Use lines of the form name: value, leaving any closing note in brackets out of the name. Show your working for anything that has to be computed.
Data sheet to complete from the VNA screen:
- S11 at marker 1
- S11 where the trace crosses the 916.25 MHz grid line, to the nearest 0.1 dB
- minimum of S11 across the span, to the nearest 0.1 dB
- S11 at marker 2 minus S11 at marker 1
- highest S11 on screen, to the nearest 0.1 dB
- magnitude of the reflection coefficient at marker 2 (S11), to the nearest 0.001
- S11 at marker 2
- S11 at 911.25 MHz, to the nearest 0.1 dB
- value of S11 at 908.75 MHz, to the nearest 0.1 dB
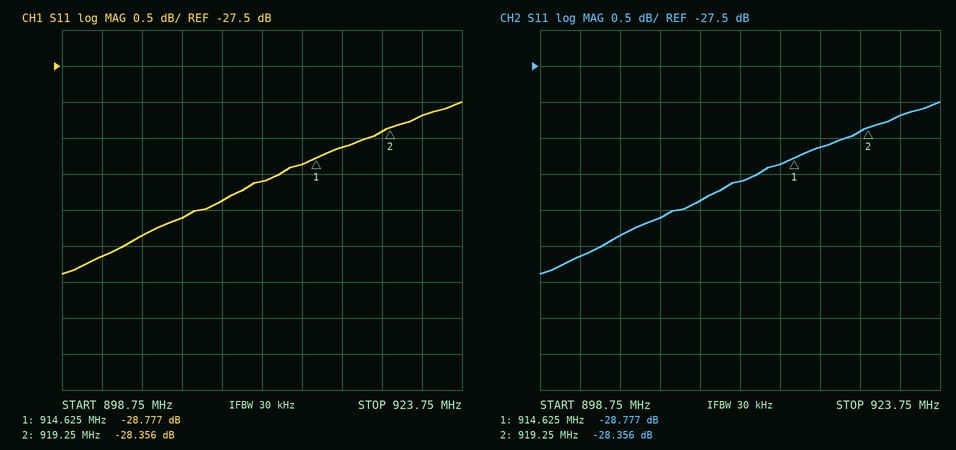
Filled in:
S11 at marker 1: -28.777 dB
S11 where the trace crosses the 916.25 MHz grid line, to the nearest 0.1 dB: -28.6 dB
minimum of S11 across the span, to the nearest 0.1 dB: -30.4 dB
S11 at marker 2 minus S11 at marker 1: -28.356 − (-28.777) = 0.421 dB
highest S11 on screen, to the nearest 0.1 dB: -28.0 dB
magnitude of the reflection coefficient at marker 2 (S11), to the nearest 0.001: 10^(-28.356/20) ≈ 0.038
S11 at marker 2: -28.356 dB
S11 at 911.25 MHz, to the nearest 0.1 dB: -29.1 dB
value of S11 at 908.75 MHz, to the nearest 0.1 dB: -29.4 dB
